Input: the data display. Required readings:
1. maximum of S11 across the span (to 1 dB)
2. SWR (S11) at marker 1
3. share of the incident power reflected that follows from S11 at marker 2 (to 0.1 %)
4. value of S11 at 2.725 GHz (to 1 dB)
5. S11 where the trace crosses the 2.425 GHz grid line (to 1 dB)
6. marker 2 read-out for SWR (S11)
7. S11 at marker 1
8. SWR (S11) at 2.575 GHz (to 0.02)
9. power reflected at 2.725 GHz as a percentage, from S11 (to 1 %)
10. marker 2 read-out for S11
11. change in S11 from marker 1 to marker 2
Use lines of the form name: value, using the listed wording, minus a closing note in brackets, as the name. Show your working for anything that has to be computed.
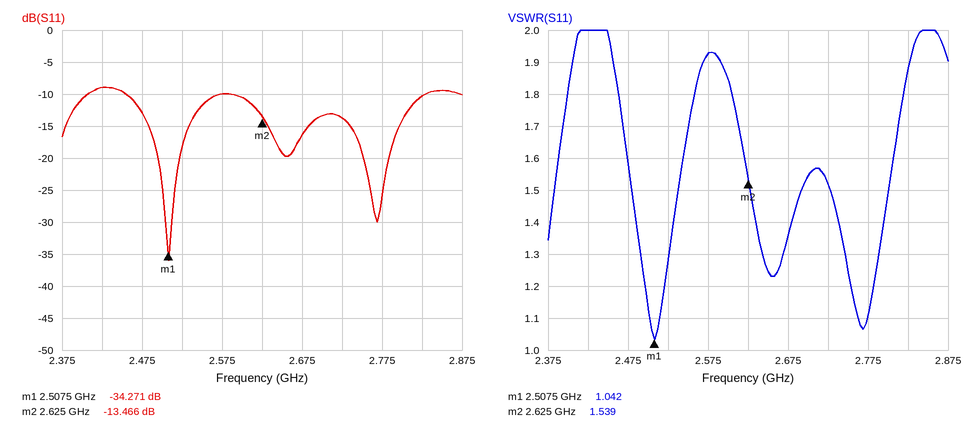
maximum of S11 across the span: -9 dB
SWR (S11) at marker 1: 1.042
share of the incident power reflected that follows from S11 at marker 2: 10^(-13.466/10) ≈ 4.5 %
value of S11 at 2.725 GHz: -14 dB
S11 where the trace crosses the 2.425 GHz grid line: -9 dB
marker 2 read-out for SWR: 1.539
S11 at marker 1: -34.271 dB
SWR (S11) at 2.575 GHz: 1.92
power reflected at 2.725 GHz as a percentage, from S11: 10^(-14/10) ≈ 4 %
marker 2 read-out for S11: -13.466 dB
change in S11 from marker 1 to marker 2: -13.466 − (-34.271) = 20.805 dB
